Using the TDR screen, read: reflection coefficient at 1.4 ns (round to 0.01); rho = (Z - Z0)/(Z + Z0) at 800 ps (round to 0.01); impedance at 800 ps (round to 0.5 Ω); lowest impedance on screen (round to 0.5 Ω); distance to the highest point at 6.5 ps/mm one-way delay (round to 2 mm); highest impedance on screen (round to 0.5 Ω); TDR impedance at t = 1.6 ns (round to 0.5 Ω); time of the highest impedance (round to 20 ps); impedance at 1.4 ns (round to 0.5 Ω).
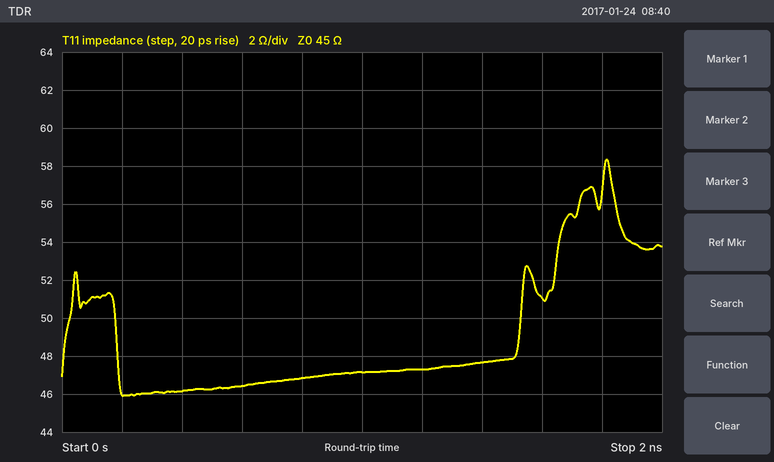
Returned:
+0.03
+0.02
47.0 Ω
46.0 Ω
140 mm
58.5 Ω
51.0 Ω
1.82 ns
47.5 Ω
